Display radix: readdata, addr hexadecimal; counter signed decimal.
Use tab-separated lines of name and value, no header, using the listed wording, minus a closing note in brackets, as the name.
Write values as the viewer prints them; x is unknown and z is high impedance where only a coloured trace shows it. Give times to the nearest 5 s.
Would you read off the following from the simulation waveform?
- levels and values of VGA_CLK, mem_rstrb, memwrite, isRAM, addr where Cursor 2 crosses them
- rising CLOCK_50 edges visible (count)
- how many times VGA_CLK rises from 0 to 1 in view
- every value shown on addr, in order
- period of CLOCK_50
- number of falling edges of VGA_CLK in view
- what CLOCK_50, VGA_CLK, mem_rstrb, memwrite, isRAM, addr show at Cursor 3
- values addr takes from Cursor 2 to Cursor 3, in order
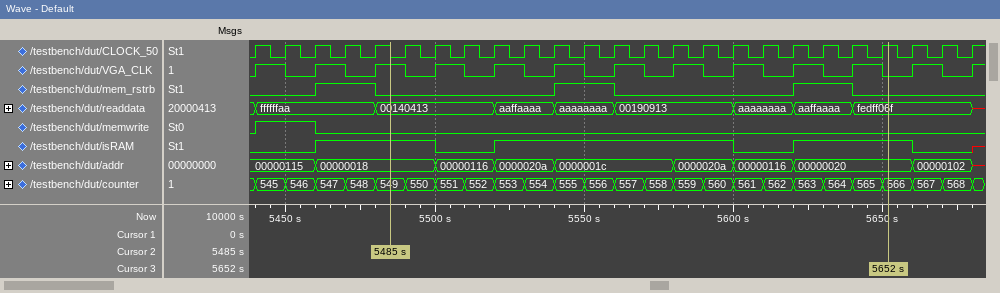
levels and values of VGA_CLK, mem_rstrb, memwrite, isRAM, addr where Cursor 2 crosses them	VGA_CLK=1, mem_rstrb=0, memwrite=0, isRAM=1, addr=00000018
rising CLOCK_50 edges visible	25
how many times VGA_CLK rises from 0 to 1 in view	13
every value shown on addr, in order	00000115, 00000018, 00000116, 0000020a, 0000001c, 0000020a, 00000116, 00000020, 00000102, x
period of CLOCK_50	10 s
number of falling edges of VGA_CLK in view	12
what CLOCK_50, VGA_CLK, mem_rstrb, memwrite, isRAM, addr show at Cursor 3	CLOCK_50=1, VGA_CLK=0, mem_rstrb=0, memwrite=0, isRAM=1, addr=00000020
values addr takes from Cursor 2 to Cursor 3, in order	00000018, 00000116, 0000020a, 0000001c, 0000020a, 00000116, 00000020
